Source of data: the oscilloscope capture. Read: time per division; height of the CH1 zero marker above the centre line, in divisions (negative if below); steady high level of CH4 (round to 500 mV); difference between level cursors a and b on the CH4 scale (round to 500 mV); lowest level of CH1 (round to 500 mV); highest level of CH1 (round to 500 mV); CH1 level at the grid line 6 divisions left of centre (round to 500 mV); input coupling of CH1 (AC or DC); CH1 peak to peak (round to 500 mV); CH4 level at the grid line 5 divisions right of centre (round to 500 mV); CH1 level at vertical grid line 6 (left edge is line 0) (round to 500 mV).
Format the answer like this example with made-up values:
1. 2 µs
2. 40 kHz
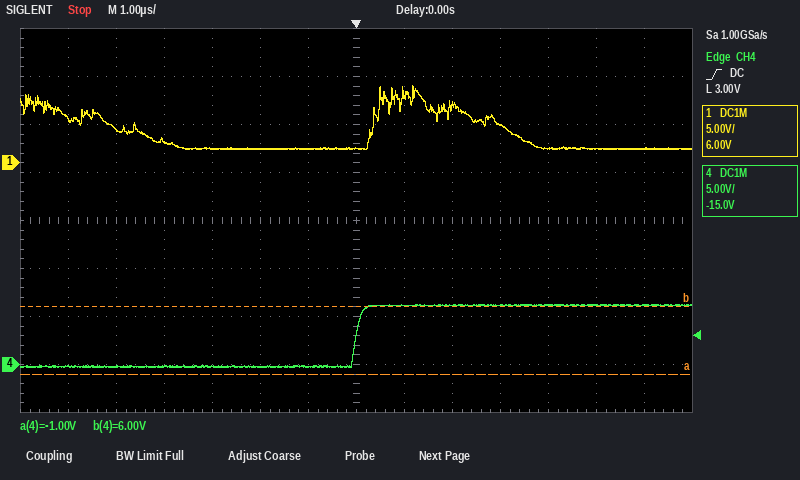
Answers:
1. 1 µs
2. +1.2 div
3. 6.0 V
4. 7.0 V
5. 1.5 V
6. 8.0 V
7. 4.5 V
8. DC
9. 6.5 V
10. 6.0 V
11. 1.5 V
